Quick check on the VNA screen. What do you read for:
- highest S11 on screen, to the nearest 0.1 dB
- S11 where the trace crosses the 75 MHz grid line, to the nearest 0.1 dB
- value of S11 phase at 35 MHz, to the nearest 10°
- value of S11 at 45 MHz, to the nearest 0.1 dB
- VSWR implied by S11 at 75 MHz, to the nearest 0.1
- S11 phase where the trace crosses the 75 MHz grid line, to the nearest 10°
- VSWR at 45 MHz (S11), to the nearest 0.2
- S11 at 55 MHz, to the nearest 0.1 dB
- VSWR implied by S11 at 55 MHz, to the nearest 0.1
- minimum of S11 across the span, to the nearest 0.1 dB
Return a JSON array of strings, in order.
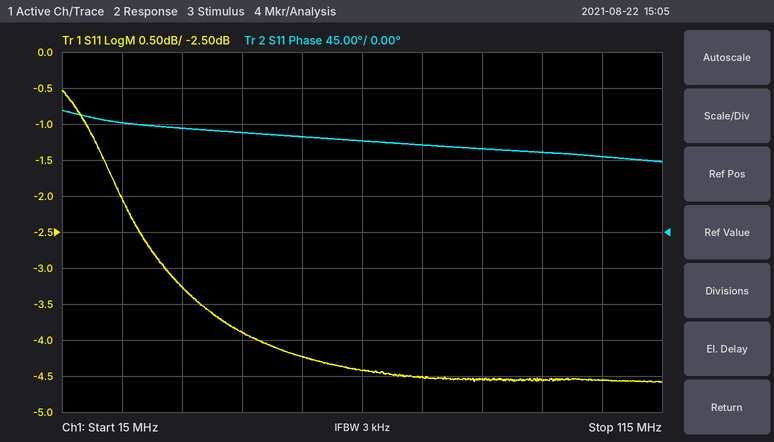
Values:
["-0.5 dB", "-4.5 dB", "130°", "-3.9 dB", "3.9", "110°", "4.6", "-4.2 dB", "4.2", "-4.6 dB"]
